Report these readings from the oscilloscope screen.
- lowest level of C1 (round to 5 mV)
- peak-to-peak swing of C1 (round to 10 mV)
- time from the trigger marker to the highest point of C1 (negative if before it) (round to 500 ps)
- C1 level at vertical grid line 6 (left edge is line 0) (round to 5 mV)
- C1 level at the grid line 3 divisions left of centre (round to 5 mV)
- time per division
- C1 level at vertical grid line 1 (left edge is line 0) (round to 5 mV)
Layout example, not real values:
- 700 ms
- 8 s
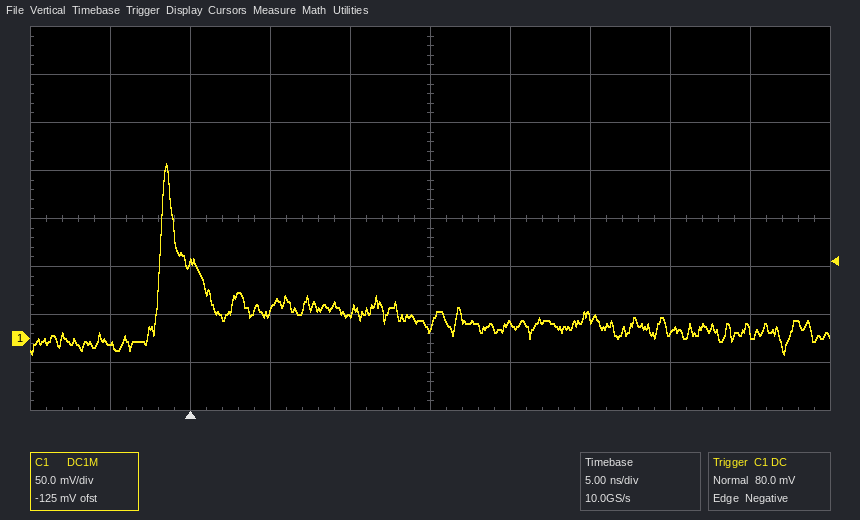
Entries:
- -15 mV
- 200 mV
- -1.5 ns
- 15 mV
- 80 mV
- 5 ns
- -5 mV
